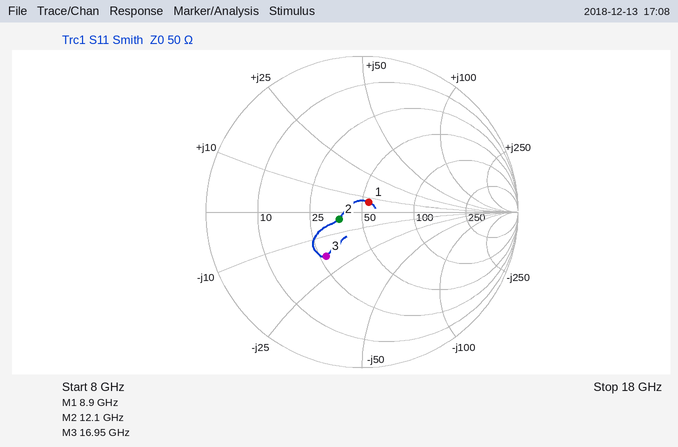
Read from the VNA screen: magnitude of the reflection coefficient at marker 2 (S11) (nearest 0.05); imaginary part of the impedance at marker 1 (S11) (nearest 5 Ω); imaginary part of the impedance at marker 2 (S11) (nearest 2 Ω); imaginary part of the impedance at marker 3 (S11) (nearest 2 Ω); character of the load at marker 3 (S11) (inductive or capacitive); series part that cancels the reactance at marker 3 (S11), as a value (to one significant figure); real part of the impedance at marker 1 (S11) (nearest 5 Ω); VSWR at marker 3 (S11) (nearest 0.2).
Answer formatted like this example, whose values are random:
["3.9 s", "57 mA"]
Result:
["0.15", "+5 Ω", "-4 Ω", "-18 Ω", "capacitive", "200 pH", "55 Ω", "2.2"]
